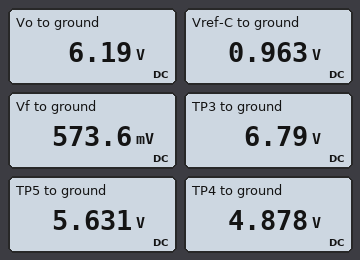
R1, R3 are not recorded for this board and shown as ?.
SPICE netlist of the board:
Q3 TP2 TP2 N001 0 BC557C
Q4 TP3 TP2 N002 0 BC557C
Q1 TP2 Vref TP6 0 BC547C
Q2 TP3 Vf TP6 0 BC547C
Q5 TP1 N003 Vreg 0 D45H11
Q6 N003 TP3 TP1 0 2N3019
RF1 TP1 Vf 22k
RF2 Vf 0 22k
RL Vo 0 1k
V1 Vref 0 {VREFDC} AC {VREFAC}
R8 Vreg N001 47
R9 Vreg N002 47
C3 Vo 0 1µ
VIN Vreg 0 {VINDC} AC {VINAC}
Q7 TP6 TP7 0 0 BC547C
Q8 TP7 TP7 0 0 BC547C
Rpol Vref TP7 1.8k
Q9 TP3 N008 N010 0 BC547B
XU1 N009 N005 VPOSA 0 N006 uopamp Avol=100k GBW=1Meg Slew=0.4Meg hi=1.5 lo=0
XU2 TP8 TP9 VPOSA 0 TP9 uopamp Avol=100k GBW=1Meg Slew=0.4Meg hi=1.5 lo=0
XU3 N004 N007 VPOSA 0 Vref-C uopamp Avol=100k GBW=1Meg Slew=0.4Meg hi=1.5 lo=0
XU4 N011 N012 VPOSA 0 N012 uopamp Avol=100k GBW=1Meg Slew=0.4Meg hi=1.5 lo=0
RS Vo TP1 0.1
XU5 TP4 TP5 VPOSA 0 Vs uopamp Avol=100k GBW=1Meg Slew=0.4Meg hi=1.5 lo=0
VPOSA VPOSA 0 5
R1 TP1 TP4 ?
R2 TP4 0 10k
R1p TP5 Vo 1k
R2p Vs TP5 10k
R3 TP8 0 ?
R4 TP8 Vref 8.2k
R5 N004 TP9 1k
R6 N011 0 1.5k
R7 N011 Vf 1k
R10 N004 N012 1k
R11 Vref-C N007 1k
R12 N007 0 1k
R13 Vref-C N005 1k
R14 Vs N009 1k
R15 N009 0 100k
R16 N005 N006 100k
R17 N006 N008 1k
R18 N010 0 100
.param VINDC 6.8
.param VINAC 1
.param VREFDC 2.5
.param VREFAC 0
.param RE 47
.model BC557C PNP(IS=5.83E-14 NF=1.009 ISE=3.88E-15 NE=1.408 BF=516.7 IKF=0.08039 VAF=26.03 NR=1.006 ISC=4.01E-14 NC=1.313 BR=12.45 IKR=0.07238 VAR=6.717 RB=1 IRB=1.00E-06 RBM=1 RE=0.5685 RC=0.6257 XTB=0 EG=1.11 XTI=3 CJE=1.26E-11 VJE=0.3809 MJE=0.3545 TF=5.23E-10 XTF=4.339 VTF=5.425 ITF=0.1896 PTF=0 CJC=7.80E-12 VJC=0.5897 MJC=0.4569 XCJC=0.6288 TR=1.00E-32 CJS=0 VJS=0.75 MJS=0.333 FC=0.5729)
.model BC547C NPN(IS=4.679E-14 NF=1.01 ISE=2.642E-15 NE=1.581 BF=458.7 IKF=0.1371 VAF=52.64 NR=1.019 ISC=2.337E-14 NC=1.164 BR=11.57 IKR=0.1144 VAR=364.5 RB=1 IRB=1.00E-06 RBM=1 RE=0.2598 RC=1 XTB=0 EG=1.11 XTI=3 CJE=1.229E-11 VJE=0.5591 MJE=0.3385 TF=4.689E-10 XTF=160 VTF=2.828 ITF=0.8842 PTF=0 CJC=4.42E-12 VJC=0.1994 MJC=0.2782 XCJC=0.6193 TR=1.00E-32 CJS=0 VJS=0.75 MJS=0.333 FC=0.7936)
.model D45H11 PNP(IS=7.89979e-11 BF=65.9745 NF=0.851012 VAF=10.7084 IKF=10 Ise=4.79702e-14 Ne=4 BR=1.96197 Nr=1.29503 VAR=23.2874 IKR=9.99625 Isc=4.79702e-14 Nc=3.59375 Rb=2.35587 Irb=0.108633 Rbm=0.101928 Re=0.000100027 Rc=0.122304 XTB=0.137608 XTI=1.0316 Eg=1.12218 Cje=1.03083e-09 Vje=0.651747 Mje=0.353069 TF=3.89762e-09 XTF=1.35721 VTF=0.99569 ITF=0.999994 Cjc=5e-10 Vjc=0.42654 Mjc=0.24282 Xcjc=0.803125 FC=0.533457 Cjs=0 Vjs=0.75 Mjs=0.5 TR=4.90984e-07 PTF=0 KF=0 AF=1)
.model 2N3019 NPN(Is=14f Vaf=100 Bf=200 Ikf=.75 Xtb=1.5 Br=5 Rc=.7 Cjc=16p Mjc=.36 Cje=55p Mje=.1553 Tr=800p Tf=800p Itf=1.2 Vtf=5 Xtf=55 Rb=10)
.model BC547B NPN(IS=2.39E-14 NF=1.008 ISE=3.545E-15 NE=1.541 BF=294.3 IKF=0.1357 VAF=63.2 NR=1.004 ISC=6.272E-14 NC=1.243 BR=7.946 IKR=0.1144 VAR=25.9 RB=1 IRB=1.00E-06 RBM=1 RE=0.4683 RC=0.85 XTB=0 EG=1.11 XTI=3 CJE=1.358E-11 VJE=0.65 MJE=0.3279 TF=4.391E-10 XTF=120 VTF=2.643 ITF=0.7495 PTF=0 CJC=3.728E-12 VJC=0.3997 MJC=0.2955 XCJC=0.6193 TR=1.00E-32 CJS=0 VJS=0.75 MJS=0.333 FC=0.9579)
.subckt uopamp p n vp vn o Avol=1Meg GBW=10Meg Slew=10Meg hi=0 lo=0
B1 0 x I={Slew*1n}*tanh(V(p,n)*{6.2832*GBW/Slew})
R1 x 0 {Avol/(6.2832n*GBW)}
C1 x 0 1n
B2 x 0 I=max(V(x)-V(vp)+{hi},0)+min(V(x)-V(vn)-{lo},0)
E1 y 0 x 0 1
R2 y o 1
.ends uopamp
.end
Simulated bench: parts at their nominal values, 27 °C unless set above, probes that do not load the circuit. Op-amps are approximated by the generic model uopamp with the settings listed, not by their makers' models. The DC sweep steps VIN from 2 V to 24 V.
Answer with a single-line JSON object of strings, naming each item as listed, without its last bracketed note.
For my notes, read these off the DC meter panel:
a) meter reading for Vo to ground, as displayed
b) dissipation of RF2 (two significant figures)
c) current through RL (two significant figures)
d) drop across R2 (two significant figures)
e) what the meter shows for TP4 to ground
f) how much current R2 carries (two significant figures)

{"meter reading for Vo to ground, as displayed": "6.19 V", "dissipation of RF2": "15 µW", "current through RL": "6.2 mA", "drop across R2": "4.9 V", "what the meter shows for TP4 to ground": "4.878 V", "how much current R2 carries": "490 µA"}
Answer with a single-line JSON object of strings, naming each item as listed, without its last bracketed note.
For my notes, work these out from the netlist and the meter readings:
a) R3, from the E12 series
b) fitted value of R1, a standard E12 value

{"R3, from the E12 series": "2.7 kΩ", "fitted value of R1, a standard E12 value": "2.7 kΩ"}
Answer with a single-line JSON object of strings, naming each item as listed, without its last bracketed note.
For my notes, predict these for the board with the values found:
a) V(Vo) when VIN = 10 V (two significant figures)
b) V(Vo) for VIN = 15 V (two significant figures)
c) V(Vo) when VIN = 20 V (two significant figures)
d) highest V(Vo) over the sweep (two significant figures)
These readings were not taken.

{"V(Vo) when VIN = 10 V": "9.4 V", "V(Vo) for VIN = 15 V": "14 V", "V(Vo) when VIN = 20 V": "19 V", "highest V(Vo) over the sweep": "23 V"}
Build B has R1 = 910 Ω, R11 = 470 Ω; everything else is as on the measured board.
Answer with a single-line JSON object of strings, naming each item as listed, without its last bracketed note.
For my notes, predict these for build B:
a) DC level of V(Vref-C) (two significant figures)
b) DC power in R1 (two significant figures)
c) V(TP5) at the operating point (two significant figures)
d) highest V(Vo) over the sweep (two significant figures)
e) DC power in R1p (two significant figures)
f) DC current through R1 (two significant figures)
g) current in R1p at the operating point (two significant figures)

{"DC level of V(Vref-C)": "710 mV", "DC power in R1": "290 µW", "V(TP5) at the operating point": "5.7 V", "highest V(Vo) over the sweep": "11 V", "DC power in R1p": "270 µW", "DC current through R1": "570 µA", "current in R1p at the operating point": "520 µA"}
